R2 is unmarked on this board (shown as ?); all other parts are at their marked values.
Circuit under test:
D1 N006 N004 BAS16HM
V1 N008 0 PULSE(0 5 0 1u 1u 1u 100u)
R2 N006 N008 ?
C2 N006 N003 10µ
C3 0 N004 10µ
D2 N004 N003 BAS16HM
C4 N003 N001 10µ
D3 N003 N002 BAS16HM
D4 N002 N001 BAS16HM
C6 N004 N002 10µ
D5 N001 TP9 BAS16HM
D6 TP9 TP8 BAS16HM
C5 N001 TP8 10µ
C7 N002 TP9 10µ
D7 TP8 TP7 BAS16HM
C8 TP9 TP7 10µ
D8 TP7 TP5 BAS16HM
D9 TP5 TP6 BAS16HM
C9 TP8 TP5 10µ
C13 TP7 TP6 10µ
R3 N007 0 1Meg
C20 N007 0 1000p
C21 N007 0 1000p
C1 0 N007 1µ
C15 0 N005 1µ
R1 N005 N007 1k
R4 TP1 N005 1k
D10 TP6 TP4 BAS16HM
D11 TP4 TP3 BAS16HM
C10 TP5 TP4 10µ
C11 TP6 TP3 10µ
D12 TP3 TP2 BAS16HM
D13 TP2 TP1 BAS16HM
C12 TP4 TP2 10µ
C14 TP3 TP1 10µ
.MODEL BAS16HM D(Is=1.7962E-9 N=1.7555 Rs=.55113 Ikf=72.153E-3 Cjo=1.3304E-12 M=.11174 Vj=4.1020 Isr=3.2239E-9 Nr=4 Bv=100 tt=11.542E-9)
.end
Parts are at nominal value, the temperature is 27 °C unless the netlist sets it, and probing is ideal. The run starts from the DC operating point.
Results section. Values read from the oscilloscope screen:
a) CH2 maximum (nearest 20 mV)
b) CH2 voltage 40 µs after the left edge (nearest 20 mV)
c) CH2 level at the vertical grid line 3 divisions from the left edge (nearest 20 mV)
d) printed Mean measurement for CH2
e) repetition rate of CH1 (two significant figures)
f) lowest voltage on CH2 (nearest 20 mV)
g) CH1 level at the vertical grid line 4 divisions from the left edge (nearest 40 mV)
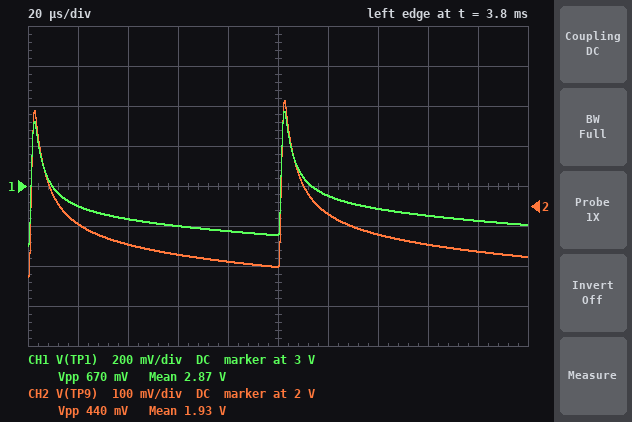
2.26 V
1.90 V
1.88 V
1.93 V
10 kHz
1.82 V
2.76 V
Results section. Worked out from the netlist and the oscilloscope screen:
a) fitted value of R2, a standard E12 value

2.7 Ω
